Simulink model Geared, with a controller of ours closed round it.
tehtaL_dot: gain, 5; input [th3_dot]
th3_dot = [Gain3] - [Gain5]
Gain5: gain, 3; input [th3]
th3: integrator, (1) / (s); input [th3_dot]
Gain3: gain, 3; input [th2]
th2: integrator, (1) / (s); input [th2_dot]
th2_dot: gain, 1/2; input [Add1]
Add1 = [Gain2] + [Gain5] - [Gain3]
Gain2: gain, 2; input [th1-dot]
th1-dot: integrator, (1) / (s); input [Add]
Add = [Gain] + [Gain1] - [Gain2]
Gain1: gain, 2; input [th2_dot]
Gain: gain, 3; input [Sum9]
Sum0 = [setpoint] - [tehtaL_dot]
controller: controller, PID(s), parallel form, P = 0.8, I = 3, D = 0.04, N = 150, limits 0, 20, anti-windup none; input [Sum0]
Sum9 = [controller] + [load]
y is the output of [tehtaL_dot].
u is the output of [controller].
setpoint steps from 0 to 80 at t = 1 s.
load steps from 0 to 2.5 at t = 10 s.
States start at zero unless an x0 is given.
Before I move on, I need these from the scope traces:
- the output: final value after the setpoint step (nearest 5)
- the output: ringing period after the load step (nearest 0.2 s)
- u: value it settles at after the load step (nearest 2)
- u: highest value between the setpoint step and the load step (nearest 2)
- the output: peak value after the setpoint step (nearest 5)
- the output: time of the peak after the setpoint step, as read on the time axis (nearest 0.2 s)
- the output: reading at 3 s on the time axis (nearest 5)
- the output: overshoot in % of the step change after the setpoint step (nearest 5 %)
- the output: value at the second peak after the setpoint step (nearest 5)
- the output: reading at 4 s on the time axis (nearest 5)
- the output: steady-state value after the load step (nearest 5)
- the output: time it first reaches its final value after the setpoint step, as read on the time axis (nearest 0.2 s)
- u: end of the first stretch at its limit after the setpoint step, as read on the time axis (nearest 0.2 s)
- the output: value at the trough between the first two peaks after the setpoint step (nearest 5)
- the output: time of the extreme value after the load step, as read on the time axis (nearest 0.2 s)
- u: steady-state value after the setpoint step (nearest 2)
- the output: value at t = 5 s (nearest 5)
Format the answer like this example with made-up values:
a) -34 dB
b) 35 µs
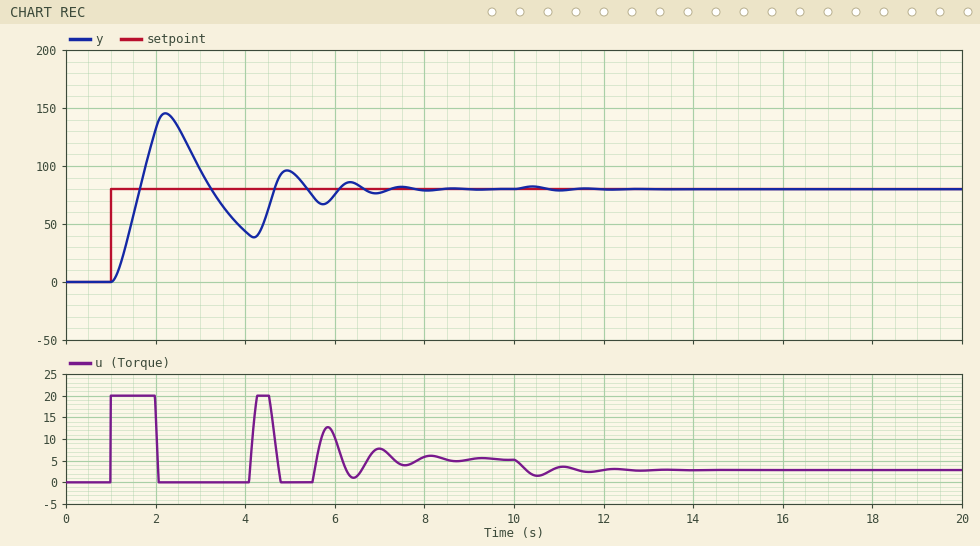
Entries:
a) 80
b) 1.2 s
c) 2
d) 20
e) 145
f) 2.2 s
g) 95
h) 80 %
i) 95
j) 45
k) 80
l) 1.6 s
m) 2.0 s
n) 40
o) 10.4 s
p) 6
q) 95
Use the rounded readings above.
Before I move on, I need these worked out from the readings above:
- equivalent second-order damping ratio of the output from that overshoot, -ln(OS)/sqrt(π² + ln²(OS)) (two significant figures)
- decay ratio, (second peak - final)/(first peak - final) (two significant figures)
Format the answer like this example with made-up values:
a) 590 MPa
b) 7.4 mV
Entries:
a) 0.071
b) 0.23
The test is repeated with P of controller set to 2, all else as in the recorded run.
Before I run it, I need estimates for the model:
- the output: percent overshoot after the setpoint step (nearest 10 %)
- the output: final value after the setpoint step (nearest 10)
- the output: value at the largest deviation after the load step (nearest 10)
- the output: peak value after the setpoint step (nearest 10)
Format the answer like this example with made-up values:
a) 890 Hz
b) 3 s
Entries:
a) 60 %
b) 80
c) 80
d) 130
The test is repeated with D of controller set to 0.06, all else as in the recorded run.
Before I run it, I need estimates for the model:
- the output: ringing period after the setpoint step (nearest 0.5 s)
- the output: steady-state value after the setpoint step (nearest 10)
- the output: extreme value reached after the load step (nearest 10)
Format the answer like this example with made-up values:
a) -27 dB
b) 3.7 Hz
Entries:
a) 2.5 s
b) 80
c) 80
